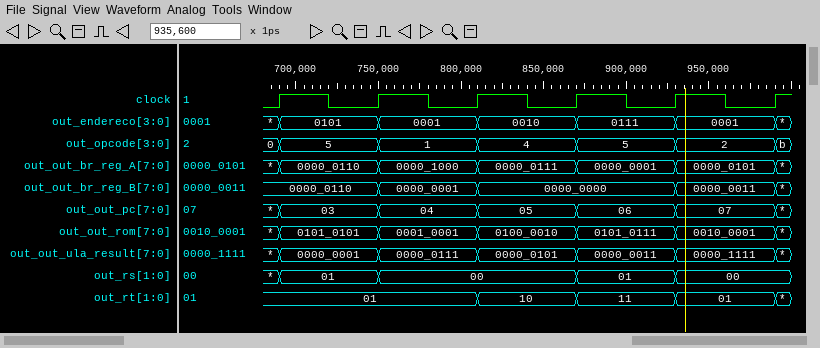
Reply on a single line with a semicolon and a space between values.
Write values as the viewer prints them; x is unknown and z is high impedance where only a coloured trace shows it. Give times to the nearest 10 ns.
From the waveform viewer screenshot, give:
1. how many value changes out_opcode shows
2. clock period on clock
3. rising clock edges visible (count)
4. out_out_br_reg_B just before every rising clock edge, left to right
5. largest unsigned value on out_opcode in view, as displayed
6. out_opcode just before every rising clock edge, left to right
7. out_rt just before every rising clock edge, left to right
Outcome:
6; 60 ns; 6; 0000_0110, 0000_0110, 0000_0001, 0000_0000, 0000_0000, 0000_0011; b; 0, 5, 1, 4, 5, 2; 01, 01, 01, 10, 11, 01
